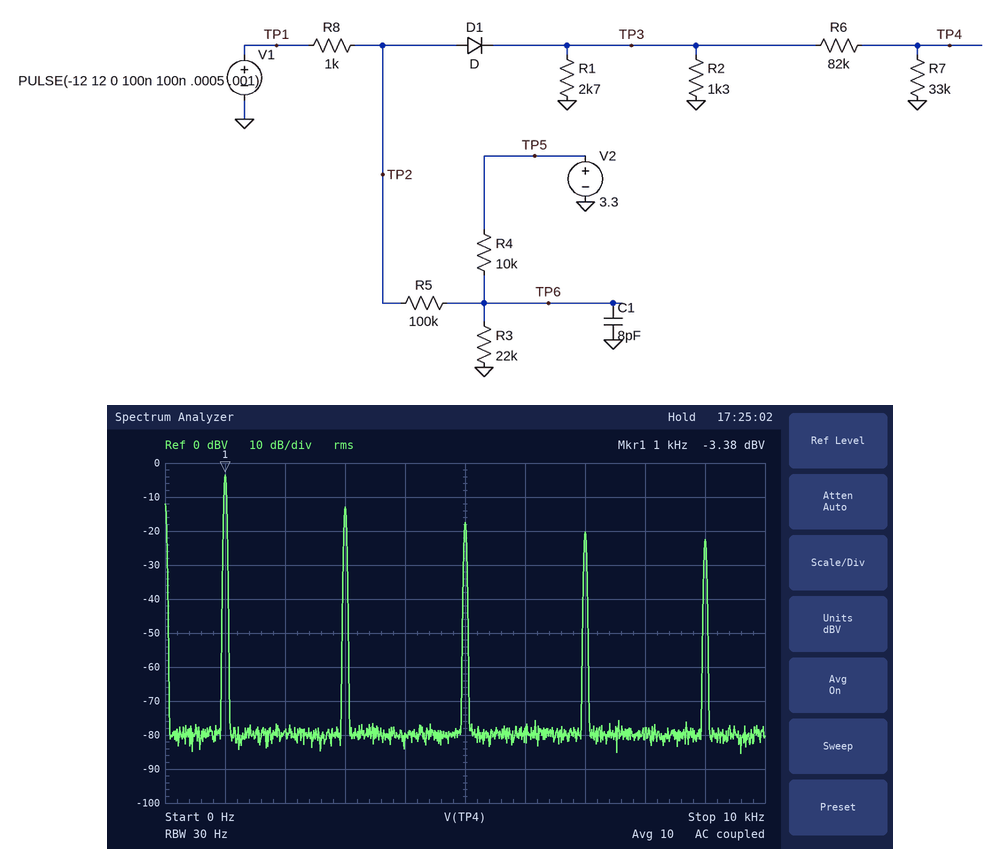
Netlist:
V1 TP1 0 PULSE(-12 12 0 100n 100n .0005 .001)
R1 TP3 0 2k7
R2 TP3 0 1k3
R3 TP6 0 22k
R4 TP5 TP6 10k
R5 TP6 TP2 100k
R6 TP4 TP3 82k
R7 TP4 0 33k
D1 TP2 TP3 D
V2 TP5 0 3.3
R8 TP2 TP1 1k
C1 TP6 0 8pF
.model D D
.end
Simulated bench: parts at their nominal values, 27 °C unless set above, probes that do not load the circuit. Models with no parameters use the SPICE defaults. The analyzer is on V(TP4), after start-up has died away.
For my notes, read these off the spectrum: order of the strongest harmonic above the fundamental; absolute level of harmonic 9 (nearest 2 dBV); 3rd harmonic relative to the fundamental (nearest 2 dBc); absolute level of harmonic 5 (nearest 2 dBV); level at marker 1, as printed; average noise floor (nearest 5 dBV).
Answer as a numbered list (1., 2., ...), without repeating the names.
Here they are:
1. 3
2. -22 dBV
3. -10 dBc
4. -18 dBV
5. -3.38 dBV
6. -80 dBV
